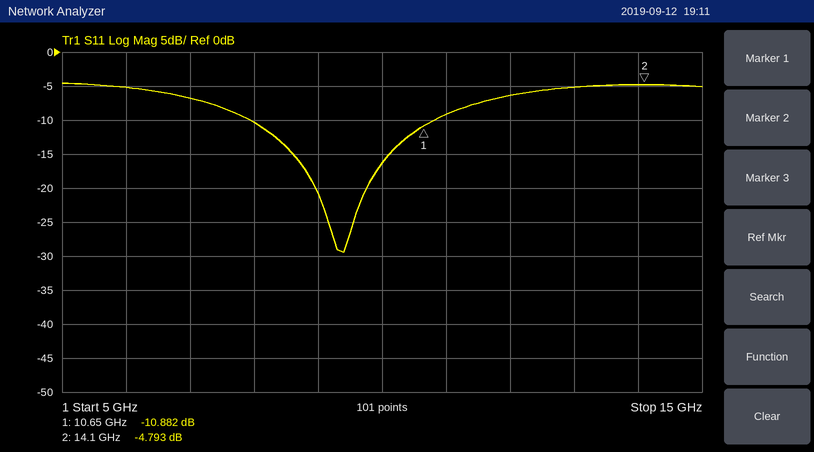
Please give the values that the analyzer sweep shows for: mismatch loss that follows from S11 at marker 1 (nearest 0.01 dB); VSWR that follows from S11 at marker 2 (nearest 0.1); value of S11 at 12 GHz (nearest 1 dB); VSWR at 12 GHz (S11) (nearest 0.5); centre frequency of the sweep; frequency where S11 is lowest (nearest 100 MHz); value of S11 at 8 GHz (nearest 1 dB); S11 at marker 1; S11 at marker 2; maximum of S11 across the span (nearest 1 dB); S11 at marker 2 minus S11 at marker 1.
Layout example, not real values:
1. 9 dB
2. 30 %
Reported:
1. 0.37 dB
2. 3.7
3. -6 dB
4. 3.0
5. 10 GHz
6. 9.4 GHz
7. -10 dB
8. -10.882 dB
9. -4.793 dB
10. -5 dB
11. 6.089 dB
